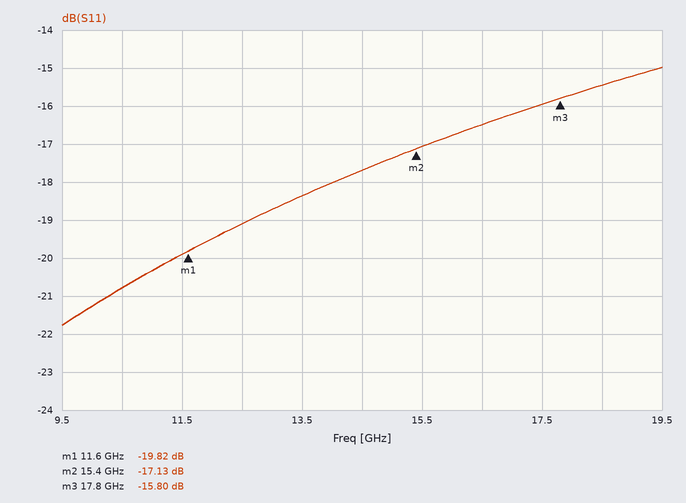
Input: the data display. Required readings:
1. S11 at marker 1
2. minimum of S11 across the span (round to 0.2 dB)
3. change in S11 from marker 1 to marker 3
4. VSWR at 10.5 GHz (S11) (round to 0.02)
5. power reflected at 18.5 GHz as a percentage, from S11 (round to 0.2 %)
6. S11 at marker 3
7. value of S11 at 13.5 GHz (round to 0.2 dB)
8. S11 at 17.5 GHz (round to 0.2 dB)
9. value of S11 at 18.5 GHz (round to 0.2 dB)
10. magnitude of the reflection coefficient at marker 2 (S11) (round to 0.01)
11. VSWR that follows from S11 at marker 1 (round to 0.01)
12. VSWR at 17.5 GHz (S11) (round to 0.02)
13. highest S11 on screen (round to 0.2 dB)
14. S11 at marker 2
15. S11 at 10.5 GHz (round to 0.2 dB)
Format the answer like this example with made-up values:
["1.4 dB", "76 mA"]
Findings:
["-19.82 dB", "-21.8 dB", "4.02 dB", "1.20", "2.8 %", "-15.80 dB", "-18.4 dB", "-16.0 dB", "-15.4 dB", "0.14", "1.23", "1.38", "-15.0 dB", "-17.13 dB", "-20.8 dB"]
